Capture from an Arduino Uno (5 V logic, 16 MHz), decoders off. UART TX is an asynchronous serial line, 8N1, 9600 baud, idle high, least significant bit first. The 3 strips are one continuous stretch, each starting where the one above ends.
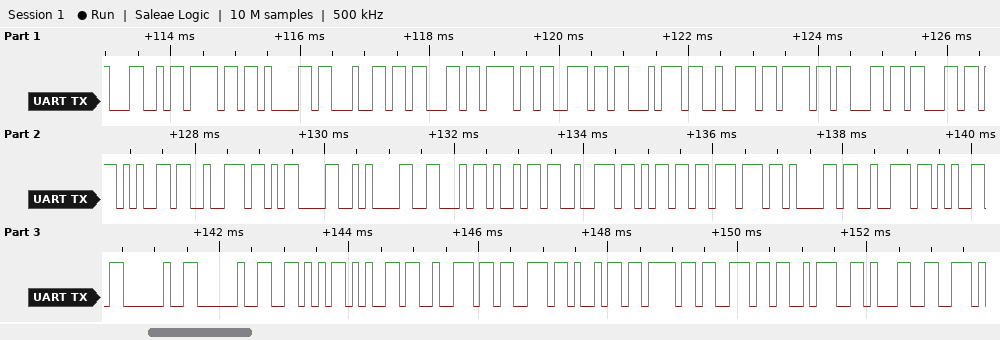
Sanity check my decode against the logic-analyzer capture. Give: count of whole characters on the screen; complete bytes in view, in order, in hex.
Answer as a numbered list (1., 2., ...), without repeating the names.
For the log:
1. 35
2. 0x4C 0x6F 0x61 0x64 0x63 0x6F 0x6E 0x74 0x72 0x6F 0x6C 0x6C 0x65 0x72 0x0D 0x0A 0x46 0x69 0x72 0x6D 0x77 0x61 0x72 0x65 0x20 0x20 0x56 0x65 0x72 0x73 0x69 0x6F 0x6E 0x3A 0x31
